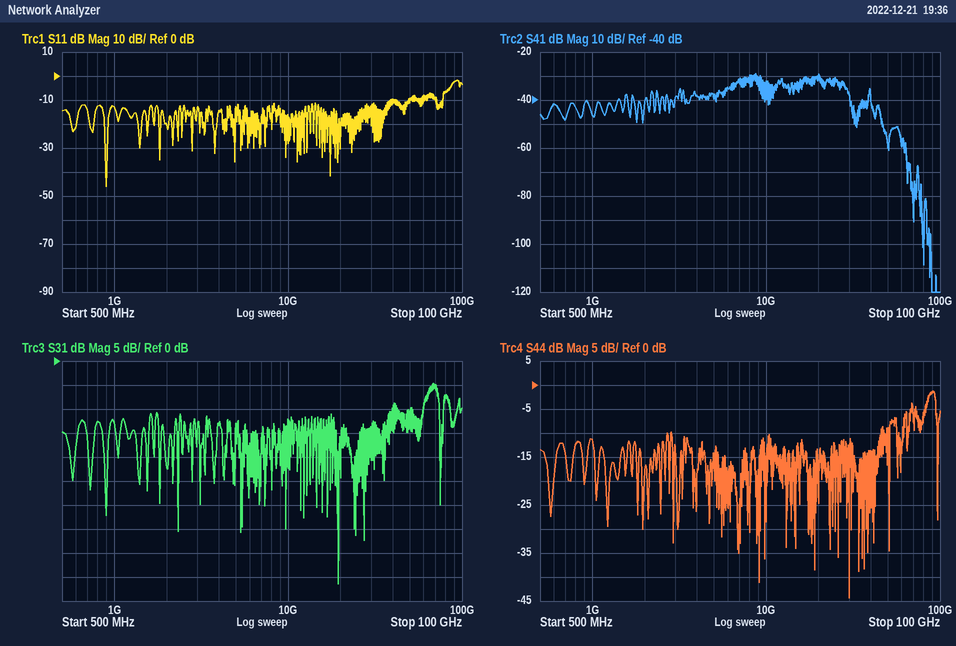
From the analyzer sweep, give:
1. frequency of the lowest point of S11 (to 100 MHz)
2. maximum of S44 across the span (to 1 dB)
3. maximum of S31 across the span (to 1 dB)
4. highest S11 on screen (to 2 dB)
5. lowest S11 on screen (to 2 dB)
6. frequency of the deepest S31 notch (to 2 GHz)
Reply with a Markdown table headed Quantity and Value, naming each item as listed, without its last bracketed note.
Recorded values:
| Quantity | Value |
|---|---|
| frequency of the lowest point of S11 | 900 MHz |
| maximum of S44 across the span | -1 dB |
| maximum of S31 across the span | -5 dB |
| highest S11 on screen | -2 dB |
| lowest S11 on screen | -46 dB |
| frequency of the deepest S31 notch | 20 GHz |
